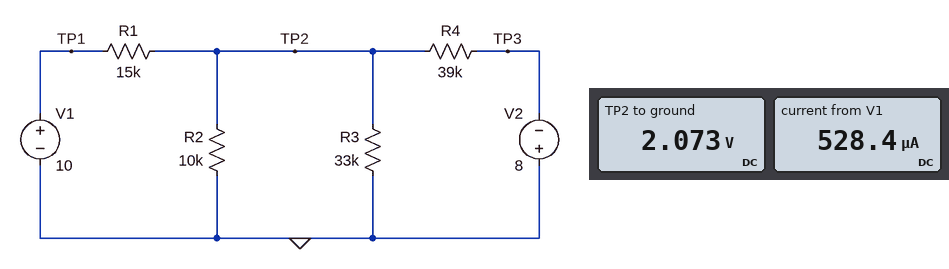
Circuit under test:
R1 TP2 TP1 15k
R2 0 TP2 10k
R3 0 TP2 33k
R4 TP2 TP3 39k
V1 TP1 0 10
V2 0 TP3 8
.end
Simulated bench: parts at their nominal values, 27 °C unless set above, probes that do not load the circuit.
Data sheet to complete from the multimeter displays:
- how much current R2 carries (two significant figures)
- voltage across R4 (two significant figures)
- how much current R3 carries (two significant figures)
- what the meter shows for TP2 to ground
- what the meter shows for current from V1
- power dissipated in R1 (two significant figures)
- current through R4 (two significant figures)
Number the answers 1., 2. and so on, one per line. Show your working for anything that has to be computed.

1. (2.073 V) / 10 kΩ = 210 µA
2. 2.073 V - (-8 V) = 10 V
3. (2.073 V) / 33 kΩ = 63 µA
4. 2.073 V
5. 528.4 µA
6. (10 V - 2.073 V)^2 / 15 kΩ = 4.2 mW
7. (2.073 V - (-8 V)) / 39 kΩ = 260 µA
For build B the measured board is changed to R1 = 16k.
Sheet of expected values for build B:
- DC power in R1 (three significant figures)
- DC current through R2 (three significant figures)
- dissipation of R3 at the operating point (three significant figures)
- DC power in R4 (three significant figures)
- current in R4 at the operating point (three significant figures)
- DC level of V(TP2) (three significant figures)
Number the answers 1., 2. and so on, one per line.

1. 4.08 mW
2. 192 µA
3. 112 µW
4. 2.52 mW
5. 254 µA
6. 1.92 V
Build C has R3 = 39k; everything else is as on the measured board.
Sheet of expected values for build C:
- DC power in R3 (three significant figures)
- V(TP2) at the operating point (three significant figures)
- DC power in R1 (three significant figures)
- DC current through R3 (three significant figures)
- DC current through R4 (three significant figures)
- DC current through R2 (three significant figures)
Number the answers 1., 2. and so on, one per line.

1. 115 µW
2. 2.12 V
3. 4.14 mW
4. 54.3 µA
5. 259 µA
6. 212 µA
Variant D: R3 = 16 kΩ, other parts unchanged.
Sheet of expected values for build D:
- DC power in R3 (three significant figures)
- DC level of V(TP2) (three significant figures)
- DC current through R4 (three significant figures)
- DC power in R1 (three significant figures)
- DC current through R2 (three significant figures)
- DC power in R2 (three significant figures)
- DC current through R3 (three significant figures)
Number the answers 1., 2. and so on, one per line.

1. 205 µW
2. 1.81 V
3. 252 µA
4. 4.47 mW
5. 181 µA
6. 328 µW
7. 113 µA
